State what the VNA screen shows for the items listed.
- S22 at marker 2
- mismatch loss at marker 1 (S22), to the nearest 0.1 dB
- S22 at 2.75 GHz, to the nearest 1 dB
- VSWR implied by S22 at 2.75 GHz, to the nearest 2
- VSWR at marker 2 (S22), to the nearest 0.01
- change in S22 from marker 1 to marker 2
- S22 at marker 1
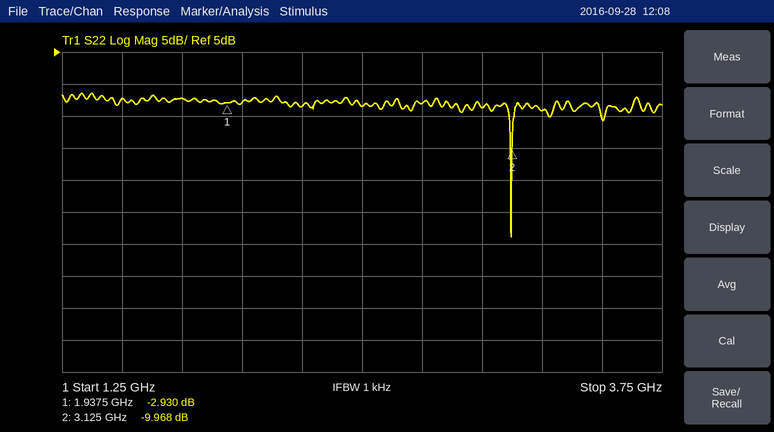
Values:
-9.968 dB
3.1 dB
-3 dB
6
1.93
-7.038 dB
-2.930 dB
